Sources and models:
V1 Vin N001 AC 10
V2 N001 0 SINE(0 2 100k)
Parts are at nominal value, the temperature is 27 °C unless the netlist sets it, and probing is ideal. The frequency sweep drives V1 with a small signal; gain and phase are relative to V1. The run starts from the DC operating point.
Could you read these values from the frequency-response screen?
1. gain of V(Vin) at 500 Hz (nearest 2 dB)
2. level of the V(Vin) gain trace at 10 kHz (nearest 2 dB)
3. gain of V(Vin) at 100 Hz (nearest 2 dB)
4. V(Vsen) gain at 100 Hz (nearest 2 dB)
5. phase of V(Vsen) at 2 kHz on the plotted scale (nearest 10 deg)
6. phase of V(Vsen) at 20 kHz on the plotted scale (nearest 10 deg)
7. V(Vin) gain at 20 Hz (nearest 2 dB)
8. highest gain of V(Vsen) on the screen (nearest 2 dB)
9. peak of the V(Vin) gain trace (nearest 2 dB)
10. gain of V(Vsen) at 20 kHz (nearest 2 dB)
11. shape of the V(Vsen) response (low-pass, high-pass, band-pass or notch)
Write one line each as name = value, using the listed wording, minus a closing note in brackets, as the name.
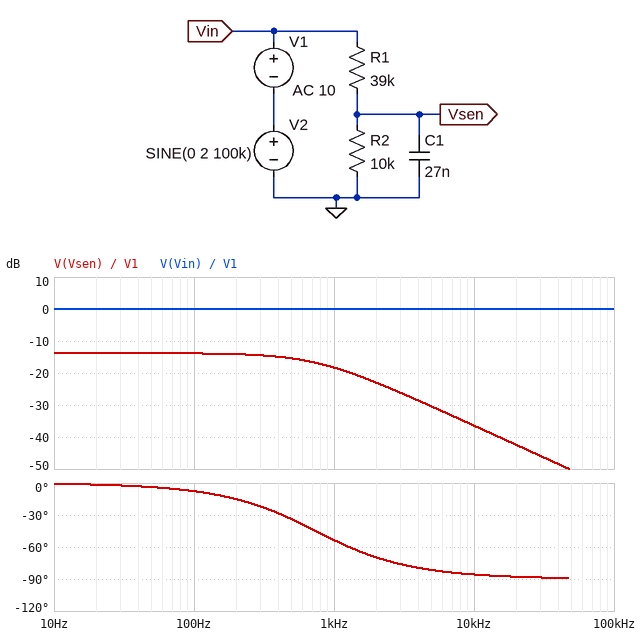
gain of V(Vin) at 500 Hz = 0 dB
level of the V(Vin) gain trace at 10 kHz = 0 dB
gain of V(Vin) at 100 Hz = 0 dB
V(Vsen) gain at 100 Hz = -14 dB
phase of V(Vsen) at 2 kHz on the plotted scale = -70 deg
phase of V(Vsen) at 20 kHz on the plotted scale = -90 deg
V(Vin) gain at 20 Hz = 0 dB
highest gain of V(Vsen) on the screen = -14 dB
peak of the V(Vin) gain trace = 0 dB
gain of V(Vsen) at 20 kHz = -42 dB
shape of the V(Vsen) response = low-pass
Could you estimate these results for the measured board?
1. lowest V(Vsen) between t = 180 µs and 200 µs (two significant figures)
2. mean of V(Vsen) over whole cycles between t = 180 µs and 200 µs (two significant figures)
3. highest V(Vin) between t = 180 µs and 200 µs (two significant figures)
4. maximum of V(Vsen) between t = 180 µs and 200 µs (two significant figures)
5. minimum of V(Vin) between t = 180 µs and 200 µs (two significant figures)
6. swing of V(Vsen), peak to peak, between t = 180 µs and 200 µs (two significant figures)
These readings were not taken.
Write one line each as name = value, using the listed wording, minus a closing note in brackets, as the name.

lowest V(Vsen) between t = 180 µs and 200 µs = -1.8 mV
mean of V(Vsen) over whole cycles between t = 180 µs and 200 µs = 1.3 mV
highest V(Vin) between t = 180 µs and 200 µs = 2.0 V
maximum of V(Vsen) between t = 180 µs and 200 µs = 4.3 mV
minimum of V(Vin) between t = 180 µs and 200 µs = -2.0 V
swing of V(Vsen), peak to peak, between t = 180 µs and 200 µs = 6.1 mV
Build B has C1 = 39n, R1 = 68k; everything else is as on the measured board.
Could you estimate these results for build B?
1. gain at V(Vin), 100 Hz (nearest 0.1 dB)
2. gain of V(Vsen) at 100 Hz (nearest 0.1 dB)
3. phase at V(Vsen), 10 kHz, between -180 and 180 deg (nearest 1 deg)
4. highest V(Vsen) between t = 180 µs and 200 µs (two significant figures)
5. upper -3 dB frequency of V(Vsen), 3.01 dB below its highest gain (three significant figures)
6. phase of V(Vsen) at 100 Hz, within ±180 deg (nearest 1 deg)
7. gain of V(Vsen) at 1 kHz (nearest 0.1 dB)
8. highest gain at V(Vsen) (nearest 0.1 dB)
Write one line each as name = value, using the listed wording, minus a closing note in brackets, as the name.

gain at V(Vin), 100 Hz = 0 dB
gain of V(Vsen) at 100 Hz = -18.0 dB
phase at V(Vsen), 10 kHz, between -180 and 180 deg = -87 deg
highest V(Vsen) between t = 180 µs and 200 µs = 1.9 mV
upper -3 dB frequency of V(Vsen), 3.01 dB below its highest gain = 468 Hz
phase of V(Vsen) at 100 Hz, within ±180 deg = -12 deg
gain of V(Vsen) at 1 kHz = -25.3 dB
highest gain at V(Vsen) = -17.8 dB
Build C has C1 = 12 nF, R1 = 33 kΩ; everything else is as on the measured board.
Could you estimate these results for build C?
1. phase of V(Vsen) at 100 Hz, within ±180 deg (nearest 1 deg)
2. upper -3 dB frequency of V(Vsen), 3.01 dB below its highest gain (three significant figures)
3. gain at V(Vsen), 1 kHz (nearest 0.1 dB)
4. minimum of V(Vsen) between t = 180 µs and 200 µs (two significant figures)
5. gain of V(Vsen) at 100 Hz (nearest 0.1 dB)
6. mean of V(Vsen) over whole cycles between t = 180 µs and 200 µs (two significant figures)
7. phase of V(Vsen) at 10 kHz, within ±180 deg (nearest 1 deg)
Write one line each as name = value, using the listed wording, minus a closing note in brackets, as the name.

phase of V(Vsen) at 100 Hz, within ±180 deg = -3 deg
upper -3 dB frequency of V(Vsen), 3.01 dB below its highest gain = 1.73 kHz
gain at V(Vsen), 1 kHz = -13.9 dB
minimum of V(Vsen) between t = 180 µs and 200 µs = -7.1 mV
gain of V(Vsen) at 100 Hz = -12.7 dB
mean of V(Vsen) over whole cycles between t = 180 µs and 200 µs = 1.1 mV
phase of V(Vsen) at 10 kHz, within ±180 deg = -80 deg
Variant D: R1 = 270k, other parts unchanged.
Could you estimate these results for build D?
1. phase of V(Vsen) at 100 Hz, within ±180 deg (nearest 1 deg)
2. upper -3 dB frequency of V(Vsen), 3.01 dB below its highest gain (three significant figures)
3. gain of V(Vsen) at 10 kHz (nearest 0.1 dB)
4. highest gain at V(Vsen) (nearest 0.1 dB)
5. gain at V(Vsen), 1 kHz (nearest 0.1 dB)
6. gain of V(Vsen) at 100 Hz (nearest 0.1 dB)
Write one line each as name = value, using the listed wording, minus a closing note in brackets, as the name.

phase of V(Vsen) at 100 Hz, within ±180 deg = -9 deg
upper -3 dB frequency of V(Vsen), 3.01 dB below its highest gain = 611 Hz
gain of V(Vsen) at 10 kHz = -53.2 dB
highest gain at V(Vsen) = -28.9 dB
gain at V(Vsen), 1 kHz = -34.6 dB
gain of V(Vsen) at 100 Hz = -29.1 dB
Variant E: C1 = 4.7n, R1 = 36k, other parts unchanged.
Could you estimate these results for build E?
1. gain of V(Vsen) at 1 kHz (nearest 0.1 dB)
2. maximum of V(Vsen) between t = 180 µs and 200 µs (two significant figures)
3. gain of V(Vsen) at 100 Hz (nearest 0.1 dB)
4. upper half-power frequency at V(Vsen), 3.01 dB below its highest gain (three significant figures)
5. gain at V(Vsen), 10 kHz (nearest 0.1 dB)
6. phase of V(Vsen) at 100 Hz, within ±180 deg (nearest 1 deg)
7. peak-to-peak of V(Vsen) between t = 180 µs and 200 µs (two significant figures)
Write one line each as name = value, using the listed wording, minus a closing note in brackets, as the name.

gain of V(Vsen) at 1 kHz = -13.5 dB
maximum of V(Vsen) between t = 180 µs and 200 µs = 19 mV
gain of V(Vsen) at 100 Hz = -13.3 dB
upper half-power frequency at V(Vsen), 3.01 dB below its highest gain = 4.33 kHz
gain at V(Vsen), 10 kHz = -21.3 dB
phase of V(Vsen) at 100 Hz, within ±180 deg = -1 deg
peak-to-peak of V(Vsen) between t = 180 µs and 200 µs = 38 mV
